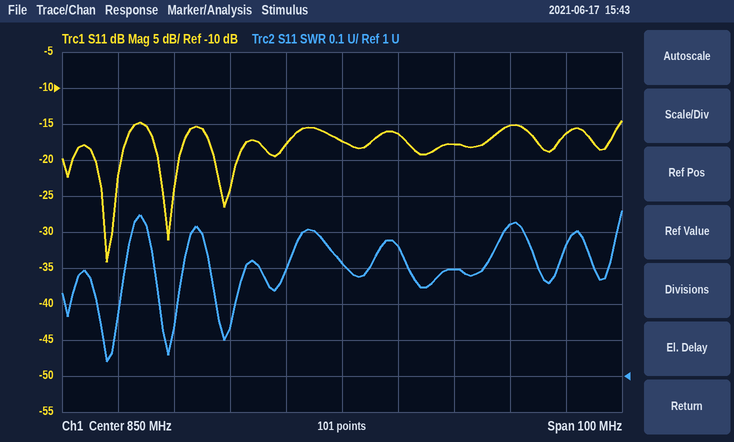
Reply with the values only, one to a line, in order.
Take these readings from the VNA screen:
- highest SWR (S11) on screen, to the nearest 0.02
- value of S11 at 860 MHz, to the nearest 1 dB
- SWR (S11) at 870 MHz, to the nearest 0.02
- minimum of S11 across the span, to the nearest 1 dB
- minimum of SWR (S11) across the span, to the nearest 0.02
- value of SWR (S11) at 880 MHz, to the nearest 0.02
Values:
1.46
-16 dB
1.30
-34 dB
1.04
1.42
